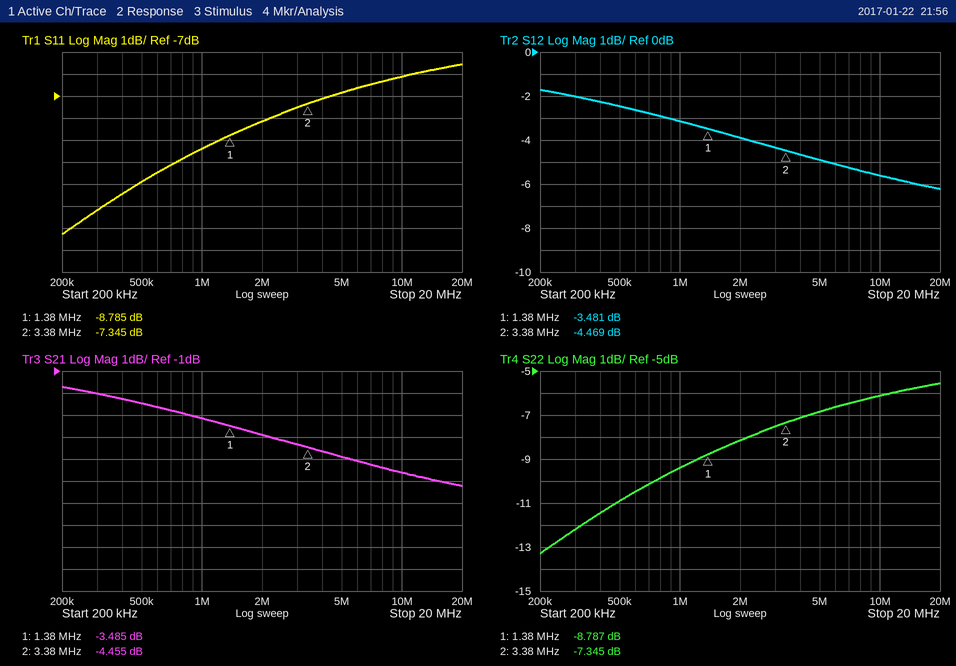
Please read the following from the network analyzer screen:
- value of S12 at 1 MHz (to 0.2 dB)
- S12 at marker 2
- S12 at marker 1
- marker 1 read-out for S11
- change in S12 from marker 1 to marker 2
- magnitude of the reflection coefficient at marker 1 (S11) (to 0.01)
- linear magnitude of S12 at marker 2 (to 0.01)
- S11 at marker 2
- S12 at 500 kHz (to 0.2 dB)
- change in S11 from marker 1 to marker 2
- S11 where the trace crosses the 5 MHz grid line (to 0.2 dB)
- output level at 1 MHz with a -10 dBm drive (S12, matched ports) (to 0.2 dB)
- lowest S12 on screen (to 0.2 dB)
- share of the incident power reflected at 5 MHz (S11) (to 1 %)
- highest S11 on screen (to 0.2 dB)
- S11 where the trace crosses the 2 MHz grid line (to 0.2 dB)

-3.2 dB
-4.469 dB
-3.481 dB
-8.785 dB
-0.988 dB
0.36
0.60
-7.345 dB
-2.4 dB
1.440 dB
-6.8 dB
-13.2 dBm
-6.2 dB
21 %
-5.6 dB
-8.2 dB
